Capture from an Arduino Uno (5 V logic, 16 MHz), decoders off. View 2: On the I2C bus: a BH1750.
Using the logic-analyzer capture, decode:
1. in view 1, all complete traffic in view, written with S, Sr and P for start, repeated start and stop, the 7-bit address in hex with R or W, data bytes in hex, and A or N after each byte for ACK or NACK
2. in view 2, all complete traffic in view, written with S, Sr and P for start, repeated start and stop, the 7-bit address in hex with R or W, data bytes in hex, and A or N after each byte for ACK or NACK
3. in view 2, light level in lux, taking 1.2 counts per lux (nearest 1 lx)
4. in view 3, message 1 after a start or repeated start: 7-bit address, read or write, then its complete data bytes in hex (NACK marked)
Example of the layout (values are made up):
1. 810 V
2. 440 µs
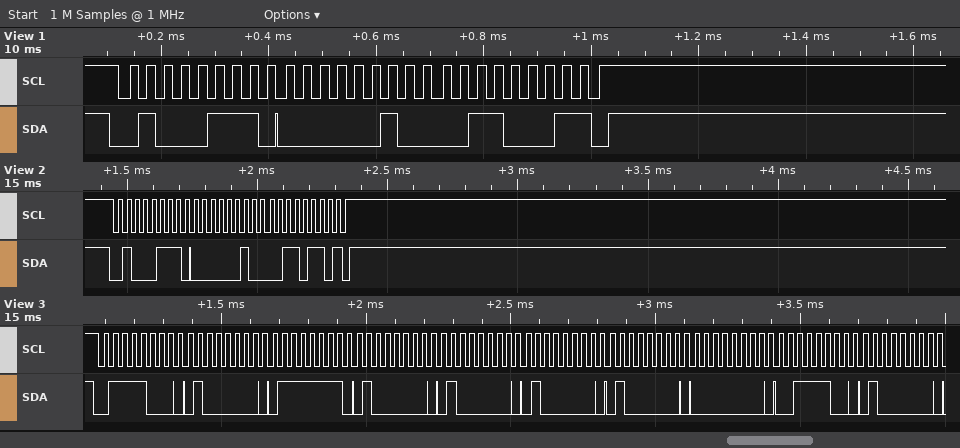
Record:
1. S 23R A 02 A 31 N P
2. S 23R A 02 A 36 N P
3. 472 lx
4. 0x3C write: 40 7F 40 40 40 40 00 3C 40
